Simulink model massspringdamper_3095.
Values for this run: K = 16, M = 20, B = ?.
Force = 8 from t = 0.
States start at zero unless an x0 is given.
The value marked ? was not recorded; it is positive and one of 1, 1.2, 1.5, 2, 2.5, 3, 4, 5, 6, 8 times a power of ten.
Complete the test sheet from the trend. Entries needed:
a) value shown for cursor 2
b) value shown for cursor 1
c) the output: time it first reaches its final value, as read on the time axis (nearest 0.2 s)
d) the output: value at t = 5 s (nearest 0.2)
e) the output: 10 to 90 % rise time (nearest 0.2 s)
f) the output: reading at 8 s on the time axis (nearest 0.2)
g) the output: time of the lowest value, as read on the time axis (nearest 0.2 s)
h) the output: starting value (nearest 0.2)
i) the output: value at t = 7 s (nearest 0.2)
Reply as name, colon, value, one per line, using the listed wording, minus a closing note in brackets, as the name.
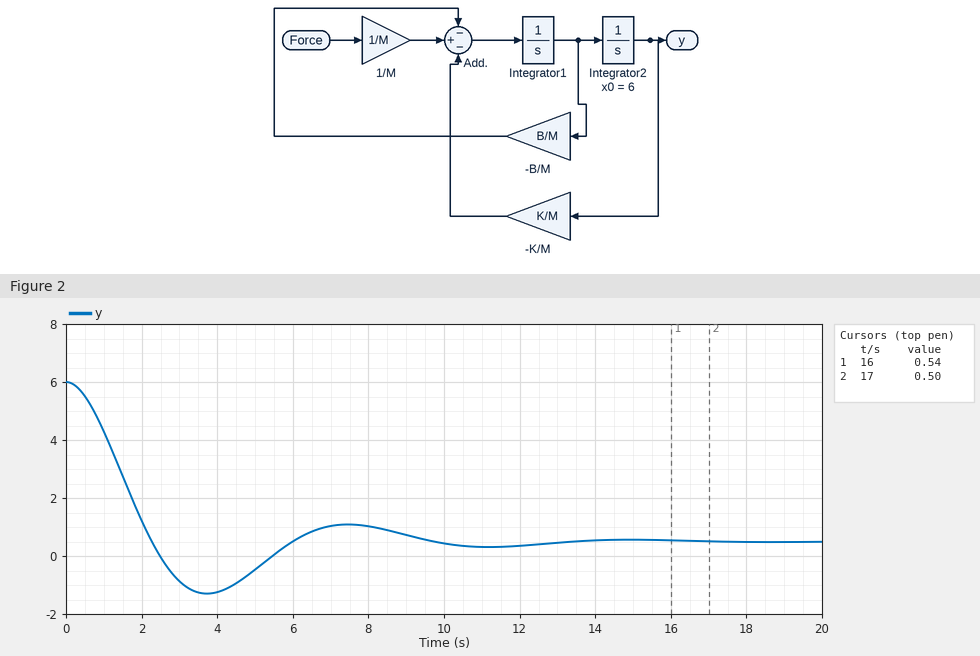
value shown for cursor 2: 0.50
value shown for cursor 1: 0.54
the output: time it first reaches its final value, as read on the time axis: 2.2 s
the output: value at t = 5 s: -0.4
the output: 10 to 90 % rise time: 1.6 s
the output: reading at 8 s on the time axis: 1.0
the output: time of the lowest value, as read on the time axis: 3.8 s
the output: starting value: 6.0
the output: value at t = 7 s: 1.0
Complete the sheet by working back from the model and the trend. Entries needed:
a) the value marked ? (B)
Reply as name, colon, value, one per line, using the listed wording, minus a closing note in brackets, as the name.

the value marked ?: 12
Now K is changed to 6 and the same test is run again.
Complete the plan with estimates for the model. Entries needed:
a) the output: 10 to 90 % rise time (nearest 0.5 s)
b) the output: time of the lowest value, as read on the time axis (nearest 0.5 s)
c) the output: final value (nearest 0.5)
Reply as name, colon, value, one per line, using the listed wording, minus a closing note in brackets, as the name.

the output: 10 to 90 % rise time: 3.0 s
the output: time of the lowest value, as read on the time axis: 7.0 s
the output: final value: 1.5
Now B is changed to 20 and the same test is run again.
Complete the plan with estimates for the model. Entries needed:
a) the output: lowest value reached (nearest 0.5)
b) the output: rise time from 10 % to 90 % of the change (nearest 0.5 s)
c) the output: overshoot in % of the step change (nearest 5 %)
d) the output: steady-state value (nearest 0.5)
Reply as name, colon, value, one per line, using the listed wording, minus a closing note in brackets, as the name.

the output: lowest value reached: 0.0
the output: rise time from 10 % to 90 % of the change: 2.0 s
the output: overshoot in % of the step change: 10 %
the output: steady-state value: 0.5
